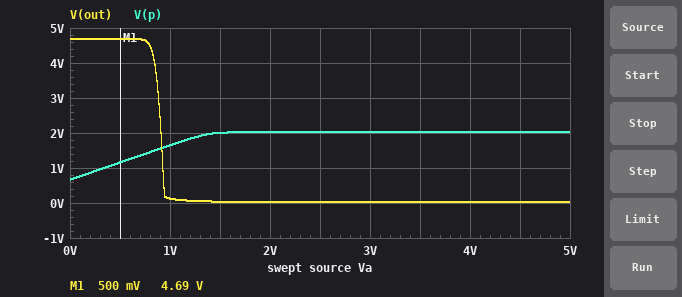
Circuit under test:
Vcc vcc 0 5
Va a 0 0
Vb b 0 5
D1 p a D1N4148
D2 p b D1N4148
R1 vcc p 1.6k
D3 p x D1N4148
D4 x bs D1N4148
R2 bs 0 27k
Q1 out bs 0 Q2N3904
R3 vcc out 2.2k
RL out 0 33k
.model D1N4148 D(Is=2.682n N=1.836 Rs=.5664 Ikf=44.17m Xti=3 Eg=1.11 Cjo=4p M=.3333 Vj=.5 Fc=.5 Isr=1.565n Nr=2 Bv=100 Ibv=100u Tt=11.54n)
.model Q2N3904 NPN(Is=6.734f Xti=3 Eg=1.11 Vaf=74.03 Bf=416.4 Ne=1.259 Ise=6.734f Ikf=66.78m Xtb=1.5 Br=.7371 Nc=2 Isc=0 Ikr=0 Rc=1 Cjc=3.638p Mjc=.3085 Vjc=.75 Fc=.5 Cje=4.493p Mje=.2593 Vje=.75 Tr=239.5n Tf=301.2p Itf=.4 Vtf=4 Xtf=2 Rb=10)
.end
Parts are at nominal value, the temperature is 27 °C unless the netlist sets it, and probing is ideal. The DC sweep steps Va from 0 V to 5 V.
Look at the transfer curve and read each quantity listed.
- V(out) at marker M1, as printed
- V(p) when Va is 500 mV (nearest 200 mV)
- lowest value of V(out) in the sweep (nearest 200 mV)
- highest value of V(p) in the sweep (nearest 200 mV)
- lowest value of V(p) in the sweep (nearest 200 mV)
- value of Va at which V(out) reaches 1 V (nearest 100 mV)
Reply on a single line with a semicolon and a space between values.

4.69 V; 1.2 V; 0 V; 2.0 V; 600 mV; 900 mV
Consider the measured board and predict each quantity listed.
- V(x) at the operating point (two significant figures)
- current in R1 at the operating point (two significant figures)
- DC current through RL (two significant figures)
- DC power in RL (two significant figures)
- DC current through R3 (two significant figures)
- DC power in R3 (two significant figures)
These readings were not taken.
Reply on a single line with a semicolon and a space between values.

360 mV; 2.7 mA; 140 µA; 670 µW; 140 µA; 44 µW
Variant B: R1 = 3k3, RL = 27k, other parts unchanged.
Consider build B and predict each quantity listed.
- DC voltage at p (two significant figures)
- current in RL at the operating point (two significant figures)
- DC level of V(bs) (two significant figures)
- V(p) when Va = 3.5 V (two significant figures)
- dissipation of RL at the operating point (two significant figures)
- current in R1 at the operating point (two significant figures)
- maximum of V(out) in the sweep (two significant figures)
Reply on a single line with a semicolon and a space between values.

630 mV; 170 µA; 42 mV; 1.9 V; 790 µW; 1.3 mA; 4.6 V
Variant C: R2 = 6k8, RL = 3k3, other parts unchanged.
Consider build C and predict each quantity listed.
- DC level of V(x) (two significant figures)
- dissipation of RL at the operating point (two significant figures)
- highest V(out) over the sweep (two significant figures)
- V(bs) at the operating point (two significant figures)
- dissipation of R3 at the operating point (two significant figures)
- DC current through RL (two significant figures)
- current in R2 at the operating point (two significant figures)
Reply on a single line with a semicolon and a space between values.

340 mV; 2.7 mW; 3.0 V; 20 mV; 1.8 mW; 910 µA; 2.9 µA
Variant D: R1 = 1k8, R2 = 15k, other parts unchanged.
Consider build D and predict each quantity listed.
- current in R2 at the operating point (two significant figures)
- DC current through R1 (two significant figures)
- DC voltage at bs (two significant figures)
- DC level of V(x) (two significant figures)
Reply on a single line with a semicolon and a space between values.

2.3 µA; 2.4 mA; 35 mV; 350 mV
